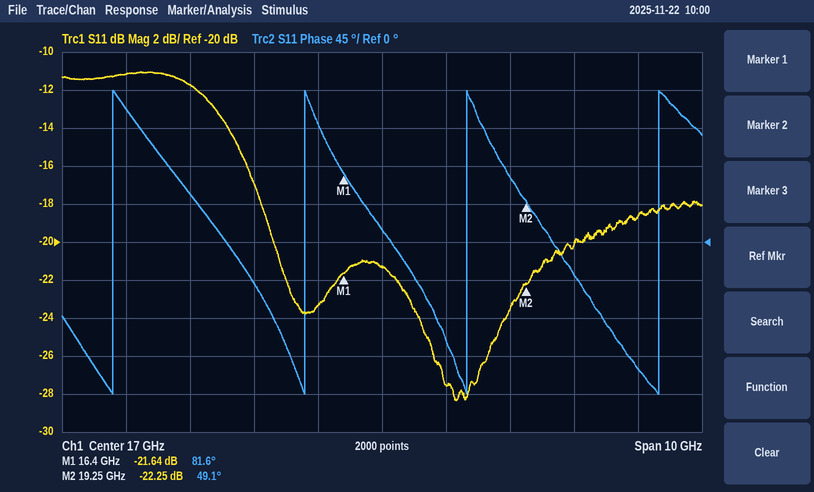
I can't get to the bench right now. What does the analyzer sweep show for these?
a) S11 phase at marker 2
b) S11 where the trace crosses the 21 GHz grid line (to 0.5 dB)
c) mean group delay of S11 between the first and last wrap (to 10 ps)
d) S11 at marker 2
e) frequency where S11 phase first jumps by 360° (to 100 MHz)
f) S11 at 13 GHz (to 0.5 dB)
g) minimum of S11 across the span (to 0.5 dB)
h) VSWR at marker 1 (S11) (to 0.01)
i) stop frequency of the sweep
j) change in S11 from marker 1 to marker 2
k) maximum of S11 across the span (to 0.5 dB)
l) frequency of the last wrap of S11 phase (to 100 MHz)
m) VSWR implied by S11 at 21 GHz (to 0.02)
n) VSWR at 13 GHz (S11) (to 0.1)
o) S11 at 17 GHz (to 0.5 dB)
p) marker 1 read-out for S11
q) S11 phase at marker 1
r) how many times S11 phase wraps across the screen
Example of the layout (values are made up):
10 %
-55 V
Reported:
49.1°
-18.5 dB
350 ps
-22.25 dB
12.8 GHz
-11.0 dB
-28.5 dB
1.18
22 GHz
-0.61 dB
-11.0 dB
21.3 GHz
1.26
1.8
-21.5 dB
-21.64 dB
81.6°
4
